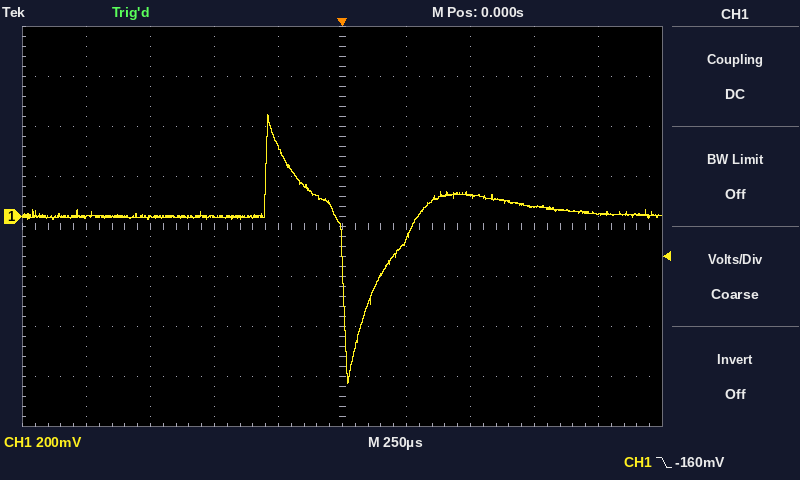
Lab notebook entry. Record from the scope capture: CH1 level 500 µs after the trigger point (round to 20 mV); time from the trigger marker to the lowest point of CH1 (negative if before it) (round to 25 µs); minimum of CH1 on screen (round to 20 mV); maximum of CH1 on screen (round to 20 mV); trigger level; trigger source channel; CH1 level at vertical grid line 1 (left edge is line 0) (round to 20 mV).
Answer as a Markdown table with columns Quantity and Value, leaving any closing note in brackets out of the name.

| Quantity | Value |
|---|---|
| CH1 level 500 µs after the trigger point | 80 mV |
| time from the trigger marker to the lowest point of CH1 (negative if before it) | +25 µs |
| minimum of CH1 on screen | -660 mV |
| maximum of CH1 on screen | 400 mV |
| trigger level | -160 mV |
| trigger source channel | CH1 |
| CH1 level at vertical grid line 1 (left edge is line 0) | 0 mV |
